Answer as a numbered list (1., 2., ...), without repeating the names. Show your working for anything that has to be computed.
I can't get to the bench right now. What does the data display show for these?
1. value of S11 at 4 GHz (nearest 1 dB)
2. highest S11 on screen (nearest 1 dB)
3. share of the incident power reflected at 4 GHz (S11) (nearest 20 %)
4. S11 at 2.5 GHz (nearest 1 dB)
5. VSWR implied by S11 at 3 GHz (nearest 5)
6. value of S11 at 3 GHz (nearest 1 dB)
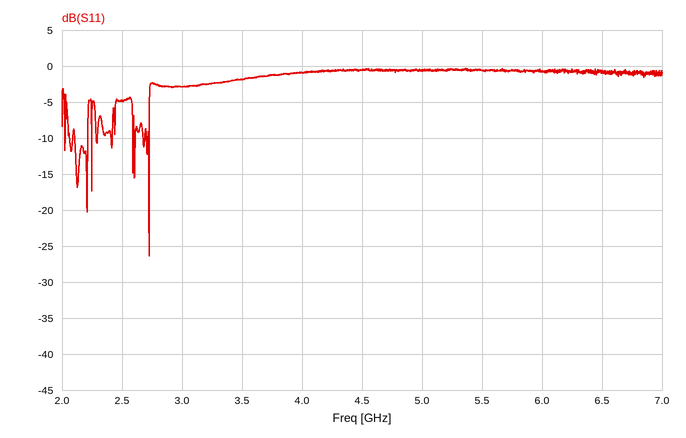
1. -1 dB
2. 0 dB
3. 10^(-1/10) ≈ 79.4 %, so 80 % to the nearest 20 %
4. -5 dB
5. |Γ| = 10^(-3/20) = 0.7079; VSWR = (1 + 0.7079)/(1 − 0.7079) ≈ 5.85, so 5 to the nearest 5
6. -3 dB
